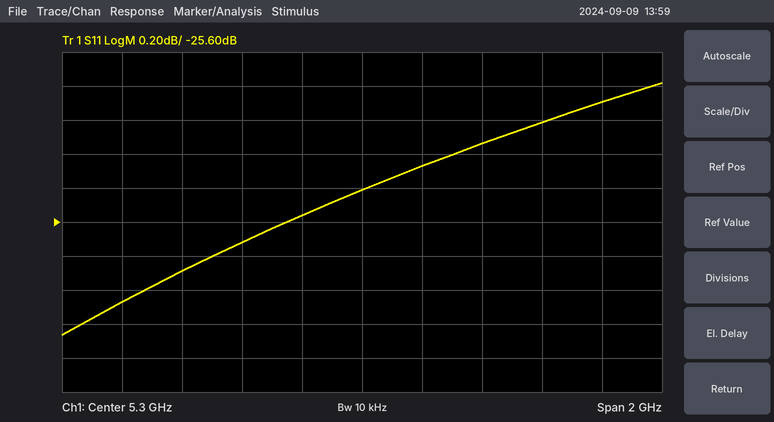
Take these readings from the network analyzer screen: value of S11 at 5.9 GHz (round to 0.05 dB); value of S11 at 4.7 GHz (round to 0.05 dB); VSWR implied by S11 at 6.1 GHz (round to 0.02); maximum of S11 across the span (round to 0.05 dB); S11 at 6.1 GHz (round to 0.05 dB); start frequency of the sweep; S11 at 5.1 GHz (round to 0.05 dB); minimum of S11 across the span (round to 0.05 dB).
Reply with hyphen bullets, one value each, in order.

- -25.00 dB
- -25.90 dB
- 1.12
- -24.80 dB
- -24.90 dB
- 4.3 GHz
- -25.55 dB
- -26.25 dB
